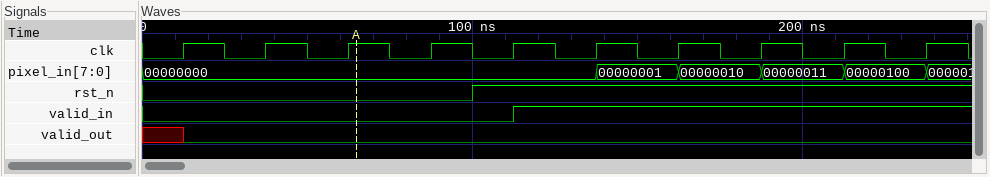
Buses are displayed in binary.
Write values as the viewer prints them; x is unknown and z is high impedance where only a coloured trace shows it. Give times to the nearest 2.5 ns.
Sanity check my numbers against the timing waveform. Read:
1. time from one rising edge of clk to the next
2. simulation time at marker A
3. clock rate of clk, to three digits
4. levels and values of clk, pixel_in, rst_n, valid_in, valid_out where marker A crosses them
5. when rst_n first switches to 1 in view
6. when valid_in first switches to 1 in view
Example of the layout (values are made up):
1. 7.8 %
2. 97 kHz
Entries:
1. 25 ns
2. 65 ns
3. 40.0 MHz
4. clk=1, pixel_in=00000000, rst_n=0, valid_in=0, valid_out=0
5. 100 ns
6. 112.5 ns
